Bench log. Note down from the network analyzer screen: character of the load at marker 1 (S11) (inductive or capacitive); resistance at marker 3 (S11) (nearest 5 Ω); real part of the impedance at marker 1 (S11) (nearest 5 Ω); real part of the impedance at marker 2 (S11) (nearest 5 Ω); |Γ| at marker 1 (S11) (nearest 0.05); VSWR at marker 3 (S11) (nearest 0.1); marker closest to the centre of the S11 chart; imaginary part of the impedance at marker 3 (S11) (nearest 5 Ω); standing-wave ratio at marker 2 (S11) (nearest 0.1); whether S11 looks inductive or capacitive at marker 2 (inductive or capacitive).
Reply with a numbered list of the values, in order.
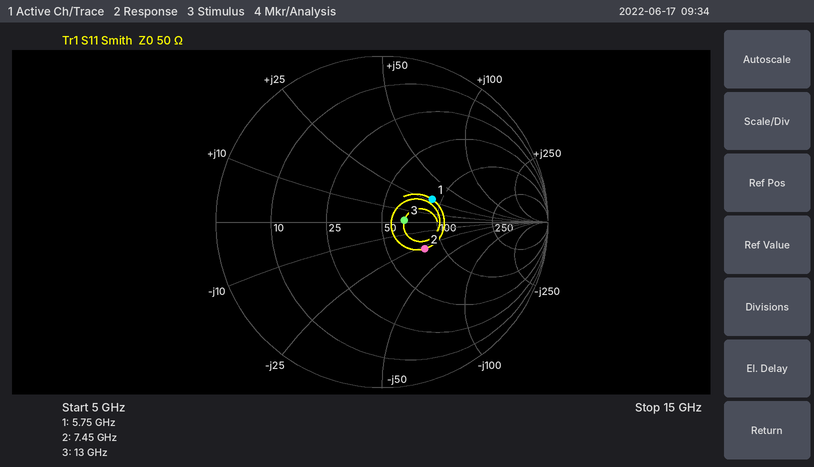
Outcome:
1. inductive
2. 65 Ω
3. 90 Ω
4. 80 Ω
5. 0.35
6. 1.3
7. marker 3
8. 0 Ω
9. 1.9
10. capacitive
